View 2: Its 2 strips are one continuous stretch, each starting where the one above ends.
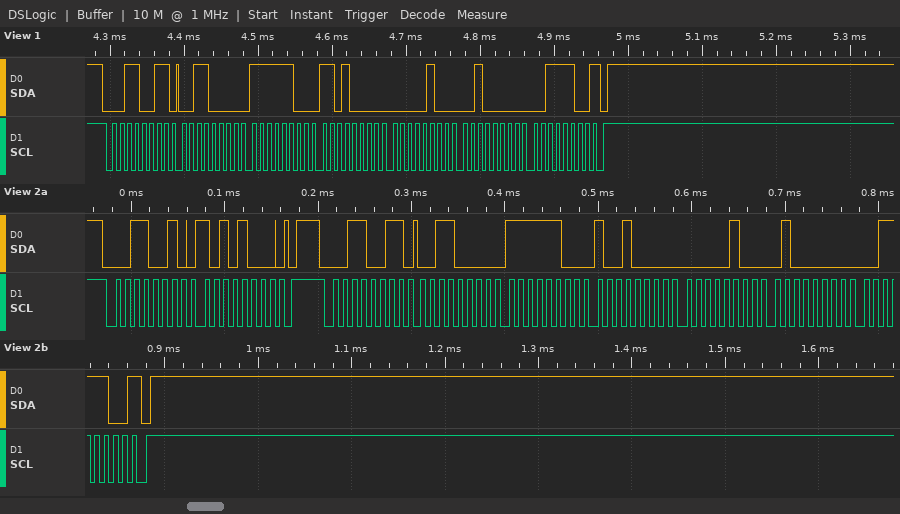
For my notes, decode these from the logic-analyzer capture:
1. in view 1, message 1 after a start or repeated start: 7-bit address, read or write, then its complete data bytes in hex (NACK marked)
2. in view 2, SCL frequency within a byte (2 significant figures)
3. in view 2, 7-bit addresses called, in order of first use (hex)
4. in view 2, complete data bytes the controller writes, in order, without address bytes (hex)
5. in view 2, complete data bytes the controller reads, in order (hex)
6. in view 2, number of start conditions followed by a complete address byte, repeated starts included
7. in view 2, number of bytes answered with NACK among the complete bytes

0x19 read: 30 FC D0 04 20 3C NACK
100 kHz
0x19
A8
30 FC 90 04 40 3C
2
1
